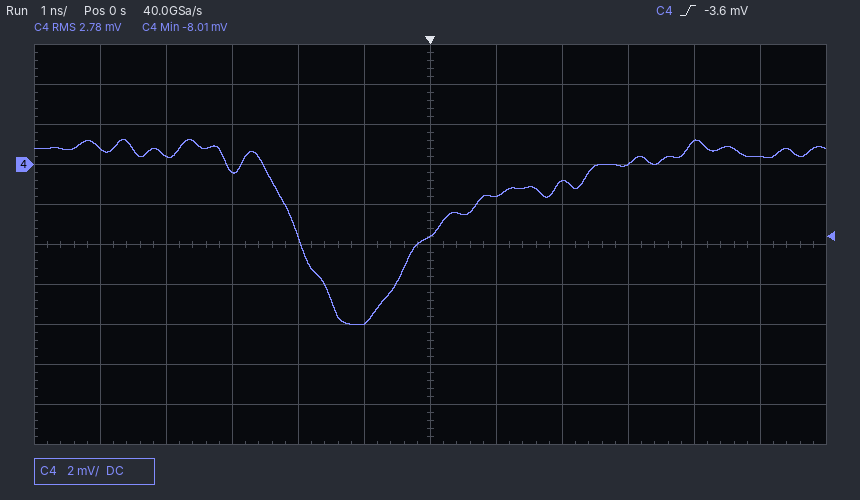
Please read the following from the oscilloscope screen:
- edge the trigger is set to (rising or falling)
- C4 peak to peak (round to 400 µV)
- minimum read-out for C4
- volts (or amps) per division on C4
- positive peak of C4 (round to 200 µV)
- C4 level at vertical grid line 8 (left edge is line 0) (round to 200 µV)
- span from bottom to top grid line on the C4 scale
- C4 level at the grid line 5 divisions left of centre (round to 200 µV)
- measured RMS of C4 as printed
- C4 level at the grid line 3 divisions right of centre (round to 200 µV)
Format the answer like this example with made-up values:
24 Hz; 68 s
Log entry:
rising; 9.2 mV; -8.01 mV; 2 mV; 1.2 mV; -800 µV; 20 mV; 800 µV; 2.78 mV; 0.0 mV
